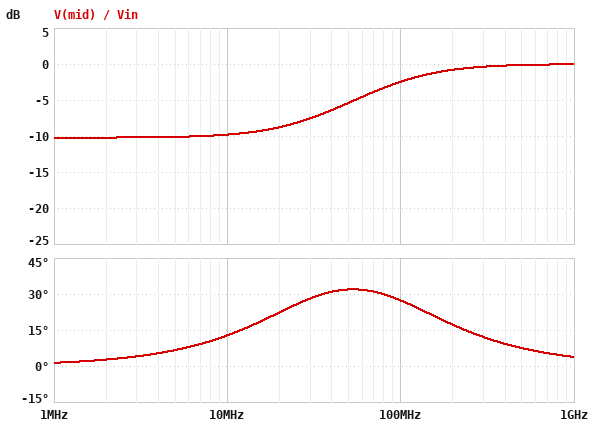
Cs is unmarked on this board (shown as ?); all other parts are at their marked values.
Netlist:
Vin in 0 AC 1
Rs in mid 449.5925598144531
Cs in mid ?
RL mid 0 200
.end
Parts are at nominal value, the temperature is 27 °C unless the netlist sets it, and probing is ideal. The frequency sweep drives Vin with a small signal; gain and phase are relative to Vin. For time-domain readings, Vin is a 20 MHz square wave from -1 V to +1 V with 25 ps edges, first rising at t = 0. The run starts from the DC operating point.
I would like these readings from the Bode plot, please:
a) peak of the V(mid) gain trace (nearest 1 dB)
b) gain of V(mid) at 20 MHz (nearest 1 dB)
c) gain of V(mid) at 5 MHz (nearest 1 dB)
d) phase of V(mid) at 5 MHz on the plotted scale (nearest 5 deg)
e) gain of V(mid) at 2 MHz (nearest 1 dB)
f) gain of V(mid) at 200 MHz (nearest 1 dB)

0 dB
-9 dB
-10 dB
5 deg
-10 dB
-1 dB
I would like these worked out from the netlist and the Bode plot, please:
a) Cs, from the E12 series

12 pF
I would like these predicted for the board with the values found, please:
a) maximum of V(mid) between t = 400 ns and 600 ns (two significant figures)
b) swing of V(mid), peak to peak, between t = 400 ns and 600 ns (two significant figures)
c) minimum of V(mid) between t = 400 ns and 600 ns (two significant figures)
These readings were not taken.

1.7 V
3.4 V
-1.7 V
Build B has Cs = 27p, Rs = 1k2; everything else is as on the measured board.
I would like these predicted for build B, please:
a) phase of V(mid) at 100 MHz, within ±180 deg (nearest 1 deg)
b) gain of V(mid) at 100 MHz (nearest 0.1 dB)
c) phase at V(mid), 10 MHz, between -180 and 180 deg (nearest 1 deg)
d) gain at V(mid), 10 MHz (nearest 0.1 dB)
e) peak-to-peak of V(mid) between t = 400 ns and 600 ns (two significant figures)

16 deg
-0.5 dB
48 deg
-10.1 dB
3.7 V
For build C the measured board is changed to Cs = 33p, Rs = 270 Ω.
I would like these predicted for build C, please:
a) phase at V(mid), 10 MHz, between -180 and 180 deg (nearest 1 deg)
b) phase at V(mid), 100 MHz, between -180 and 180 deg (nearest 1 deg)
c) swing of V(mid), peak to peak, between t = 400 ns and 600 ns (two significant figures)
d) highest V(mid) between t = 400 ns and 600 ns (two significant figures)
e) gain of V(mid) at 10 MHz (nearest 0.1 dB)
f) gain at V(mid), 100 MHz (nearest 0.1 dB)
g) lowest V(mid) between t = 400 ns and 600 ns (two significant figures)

16 deg
13 deg
3.1 V
1.6 V
-6.5 dB
-0.6 dB
-1.6 V
